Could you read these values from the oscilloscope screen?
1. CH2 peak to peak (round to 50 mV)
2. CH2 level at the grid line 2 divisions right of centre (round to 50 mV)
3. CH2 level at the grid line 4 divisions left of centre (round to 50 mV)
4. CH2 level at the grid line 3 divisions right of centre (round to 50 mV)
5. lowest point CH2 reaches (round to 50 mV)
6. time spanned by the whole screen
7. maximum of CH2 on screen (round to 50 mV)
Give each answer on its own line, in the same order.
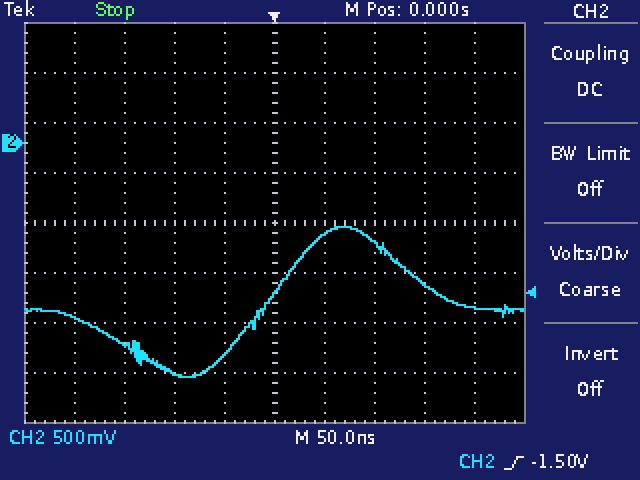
1.50 V
-1.00 V
-1.75 V
-1.40 V
-2.35 V
500 ns
-850 mV
